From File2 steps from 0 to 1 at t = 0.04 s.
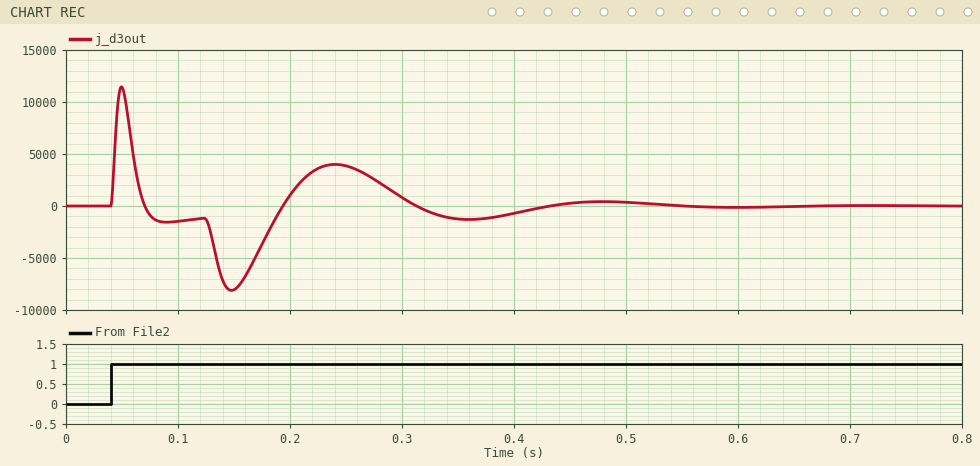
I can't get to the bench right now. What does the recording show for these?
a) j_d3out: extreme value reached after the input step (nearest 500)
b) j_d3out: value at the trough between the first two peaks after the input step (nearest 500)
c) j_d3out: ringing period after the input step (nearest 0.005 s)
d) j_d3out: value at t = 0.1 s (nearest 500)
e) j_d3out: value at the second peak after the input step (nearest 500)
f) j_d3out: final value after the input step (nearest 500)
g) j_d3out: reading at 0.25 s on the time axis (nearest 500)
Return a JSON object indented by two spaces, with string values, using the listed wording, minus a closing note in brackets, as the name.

{
  "j_d3out: extreme value reached after the input step": "11500",
  "j_d3out: value at the trough between the first two peaks after the input step": "-8000",
  "j_d3out: ringing period after the input step": "0.190 s",
  "j_d3out: value at t = 0.1 s": "-1500",
  "j_d3out: value at the second peak after the input step": "4000",
  "j_d3out: final value after the input step": "0",
  "j_d3out: reading at 0.25 s on the time axis": "4000"
}
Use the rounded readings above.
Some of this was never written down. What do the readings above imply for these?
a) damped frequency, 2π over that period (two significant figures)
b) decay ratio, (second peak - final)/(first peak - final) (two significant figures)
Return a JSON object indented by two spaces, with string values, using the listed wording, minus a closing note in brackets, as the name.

{
  "damped frequency, 2π over that period": "33 rad/s",
  "decay ratio, (second peak - final)/(first peak - final)": "0.35"
}
